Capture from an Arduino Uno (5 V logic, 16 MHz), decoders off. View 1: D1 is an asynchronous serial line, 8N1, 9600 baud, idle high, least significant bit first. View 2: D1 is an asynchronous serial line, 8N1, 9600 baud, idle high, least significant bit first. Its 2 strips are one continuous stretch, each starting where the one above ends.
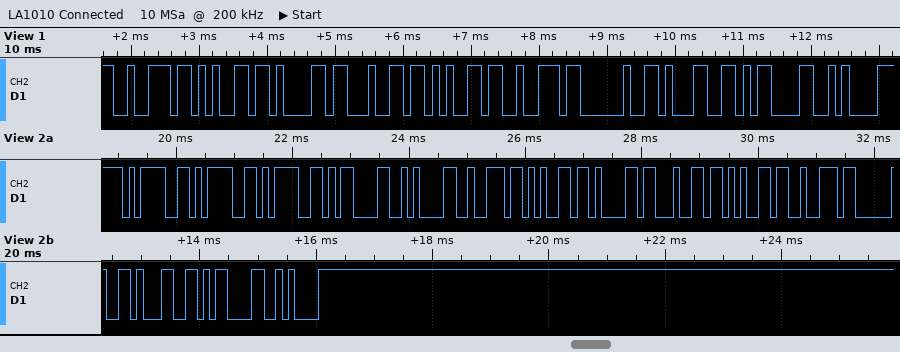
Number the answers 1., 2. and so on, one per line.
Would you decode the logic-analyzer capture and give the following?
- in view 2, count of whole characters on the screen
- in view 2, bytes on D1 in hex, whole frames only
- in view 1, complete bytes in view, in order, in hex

1. 15
2. 3D 3D 3D 0D 0A 72 65 61 64 65 72 20 31 0D 0A
3. 0x72 0x65 0x61 0x64 0x65 0x72 0x20 0x31 0x0D 0x0A
